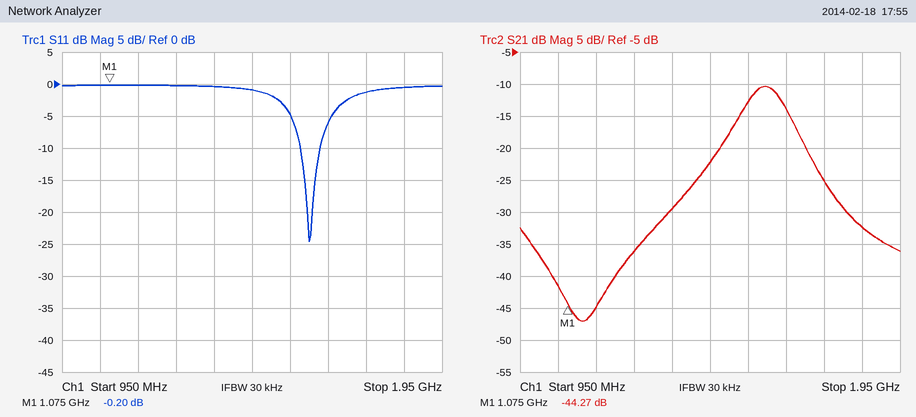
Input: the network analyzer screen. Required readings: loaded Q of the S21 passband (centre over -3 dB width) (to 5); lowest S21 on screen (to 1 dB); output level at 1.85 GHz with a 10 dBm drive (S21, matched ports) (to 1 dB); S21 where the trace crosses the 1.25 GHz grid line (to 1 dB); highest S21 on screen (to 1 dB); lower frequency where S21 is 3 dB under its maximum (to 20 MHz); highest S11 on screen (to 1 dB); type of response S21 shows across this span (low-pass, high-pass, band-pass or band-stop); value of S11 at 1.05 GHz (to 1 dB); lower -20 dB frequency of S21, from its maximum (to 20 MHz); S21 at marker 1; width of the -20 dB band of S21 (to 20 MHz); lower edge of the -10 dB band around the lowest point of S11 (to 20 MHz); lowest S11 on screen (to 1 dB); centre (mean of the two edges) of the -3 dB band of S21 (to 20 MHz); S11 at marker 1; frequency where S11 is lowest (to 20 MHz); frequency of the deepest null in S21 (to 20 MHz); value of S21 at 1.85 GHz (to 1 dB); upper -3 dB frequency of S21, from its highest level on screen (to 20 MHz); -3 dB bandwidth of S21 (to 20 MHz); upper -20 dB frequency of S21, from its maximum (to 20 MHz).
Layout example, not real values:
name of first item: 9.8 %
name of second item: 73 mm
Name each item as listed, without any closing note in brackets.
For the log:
loaded Q of the S21 passband (centre over -3 dB width): 15
lowest S21 on screen: -47 dB
output level at 1.85 GHz with a 10 dBm drive (S21, matched ports): -22 dBm
S21 where the trace crosses the 1.25 GHz grid line: -36 dB
highest S21 on screen: -10 dB
lower frequency where S21 is 3 dB under its maximum: 1.54 GHz
highest S11 on screen: 0 dB
type of response S21 shows across this span: band-pass
value of S11 at 1.05 GHz: 0 dB
lower -20 dB frequency of S21, from its maximum: 1.34 GHz
S21 at marker 1: -44.27 dB
width of the -20 dB band of S21: 480 MHz
lower edge of the -10 dB band around the lowest point of S11: 1.58 GHz
lowest S11 on screen: -25 dB
centre (mean of the two edges) of the -3 dB band of S21: 1.60 GHz
S11 at marker 1: -0.20 dB
frequency where S11 is lowest: 1.60 GHz
frequency of the deepest null in S21: 1.12 GHz
value of S21 at 1.85 GHz: -32 dB
upper -3 dB frequency of S21, from its highest level on screen: 1.64 GHz
-3 dB bandwidth of S21: 100 MHz
upper -20 dB frequency of S21, from its maximum: 1.82 GHz
